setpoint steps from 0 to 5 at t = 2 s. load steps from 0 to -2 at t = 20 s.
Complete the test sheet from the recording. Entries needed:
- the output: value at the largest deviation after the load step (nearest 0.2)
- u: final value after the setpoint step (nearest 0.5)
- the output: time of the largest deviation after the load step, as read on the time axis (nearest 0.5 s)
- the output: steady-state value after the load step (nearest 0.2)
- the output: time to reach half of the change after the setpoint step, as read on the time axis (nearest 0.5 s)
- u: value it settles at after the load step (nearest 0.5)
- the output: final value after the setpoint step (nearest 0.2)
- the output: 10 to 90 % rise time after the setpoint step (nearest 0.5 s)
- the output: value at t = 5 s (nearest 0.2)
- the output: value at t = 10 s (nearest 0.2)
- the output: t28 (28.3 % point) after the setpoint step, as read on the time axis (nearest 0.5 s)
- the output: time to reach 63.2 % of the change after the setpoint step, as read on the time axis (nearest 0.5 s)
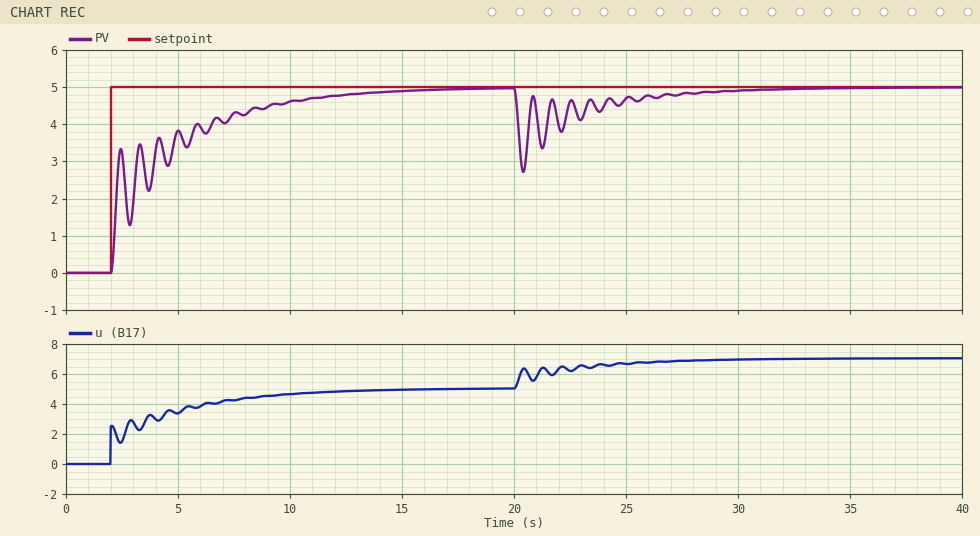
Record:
2.8
5.0
20.5 s
5.0
2.5 s
7.0
5.0
7.0 s
3.8
4.6
2.0 s
2.5 s
